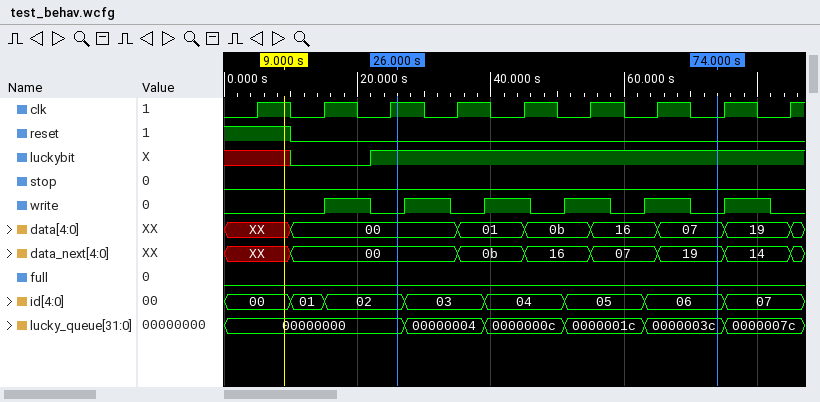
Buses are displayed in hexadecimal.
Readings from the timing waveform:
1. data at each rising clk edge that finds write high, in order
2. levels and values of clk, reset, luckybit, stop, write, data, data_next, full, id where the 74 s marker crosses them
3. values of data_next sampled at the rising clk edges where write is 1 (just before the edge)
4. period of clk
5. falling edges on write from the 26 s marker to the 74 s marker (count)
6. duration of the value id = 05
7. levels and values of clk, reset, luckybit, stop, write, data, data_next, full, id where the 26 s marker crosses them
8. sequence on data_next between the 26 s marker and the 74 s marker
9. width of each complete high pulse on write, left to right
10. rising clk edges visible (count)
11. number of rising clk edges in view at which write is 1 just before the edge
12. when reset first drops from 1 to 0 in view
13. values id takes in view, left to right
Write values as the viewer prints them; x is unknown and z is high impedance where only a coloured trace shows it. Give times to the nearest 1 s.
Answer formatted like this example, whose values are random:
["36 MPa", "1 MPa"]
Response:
["01, 0b, 16", "clk=0, reset=0, luckybit=1, stop=0, write=0, data=07, data_next=19, full=0, id=06", "0b, 16, 07", "10 s", "4", "12 s", "clk=1, reset=0, luckybit=1, stop=0, write=0, data=00, data_next=00, full=0, id=02", "00, 0b, 16, 07, 19", "7 s, 7 s, 7 s, 7 s, 7 s, 7 s", "9", "3", "10 s", "00, 01, 02, 03, 04, 05, 06, 07"]
